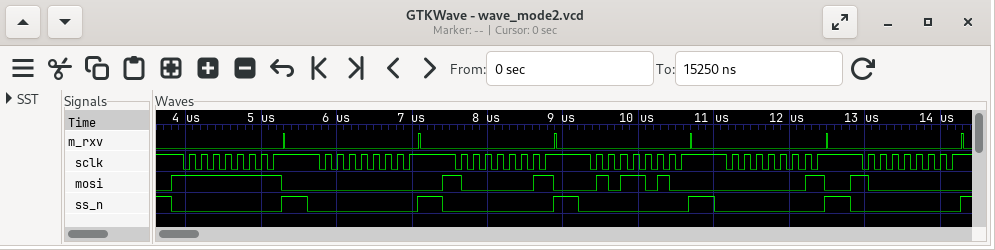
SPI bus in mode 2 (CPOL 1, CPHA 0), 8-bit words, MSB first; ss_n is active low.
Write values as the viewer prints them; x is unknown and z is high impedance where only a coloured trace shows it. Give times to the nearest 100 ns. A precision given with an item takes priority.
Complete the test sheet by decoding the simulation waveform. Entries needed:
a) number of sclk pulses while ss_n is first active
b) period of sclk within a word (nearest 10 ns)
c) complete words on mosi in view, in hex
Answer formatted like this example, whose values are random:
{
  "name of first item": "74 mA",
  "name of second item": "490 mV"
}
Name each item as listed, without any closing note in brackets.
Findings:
{
  "number of sclk pulses while ss_n is first active": "8",
  "period of sclk within a word": "160 ns",
  "complete words on mosi in view, in hex": "FF, 00, 81, 5A, 01, 80"
}
